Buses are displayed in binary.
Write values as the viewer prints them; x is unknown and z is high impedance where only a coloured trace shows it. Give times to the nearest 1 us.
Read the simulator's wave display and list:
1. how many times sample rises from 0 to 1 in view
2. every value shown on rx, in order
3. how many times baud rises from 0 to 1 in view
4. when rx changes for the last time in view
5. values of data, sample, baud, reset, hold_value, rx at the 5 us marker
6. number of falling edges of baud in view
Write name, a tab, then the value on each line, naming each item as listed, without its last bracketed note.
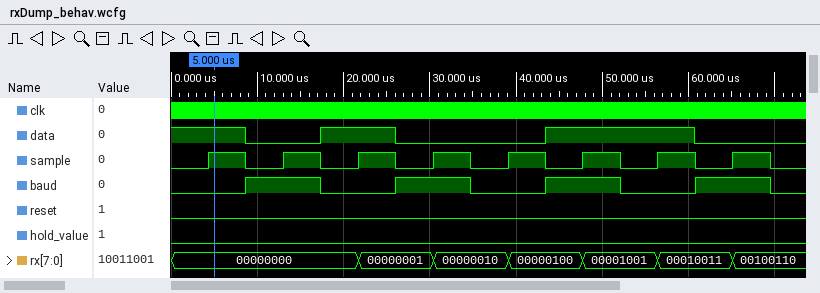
how many times sample rises from 0 to 1 in view	8
every value shown on rx, in order	00000000, 00000001, 00000010, 00000100, 00001001, 00010011, 00100110
how many times baud rises from 0 to 1 in view	4
when rx changes for the last time in view	65 us
values of data, sample, baud, reset, hold_value, rx at the 5 us marker	data=1, sample=1, baud=0, reset=0, hold_value=0, rx=00000000
number of falling edges of baud in view	4
